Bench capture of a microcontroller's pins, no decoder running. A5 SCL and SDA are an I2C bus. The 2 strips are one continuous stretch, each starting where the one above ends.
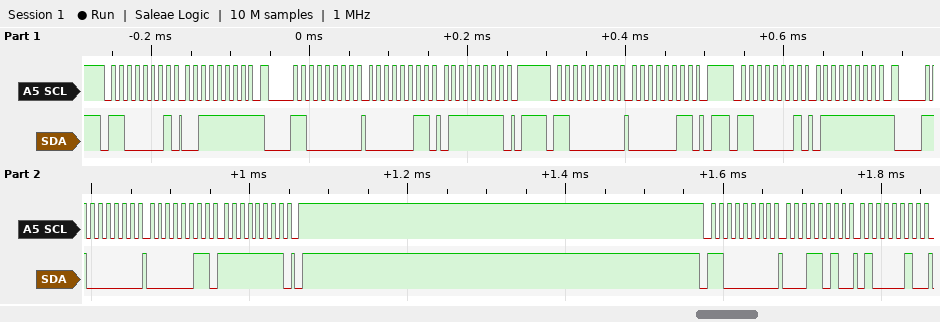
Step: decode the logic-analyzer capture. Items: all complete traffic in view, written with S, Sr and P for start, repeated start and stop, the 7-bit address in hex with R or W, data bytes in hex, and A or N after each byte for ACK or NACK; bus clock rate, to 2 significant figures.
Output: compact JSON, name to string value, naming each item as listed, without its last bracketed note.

{"all complete traffic in view, written with S, Sr and P for start, repeated start and stop, the 7-bit address in hex with R or W, data bytes in hex, and A or N after each byte for ACK or NACK": "S 60R A 3F N Sr 60W A 03 A 7F A P S 60W A 03 A P S 60R A 7F N Sr 60W A 03 A FF A P S 60W A 1A A 42 A", "bus clock rate, to 2 significant figures": "100 kHz"}
